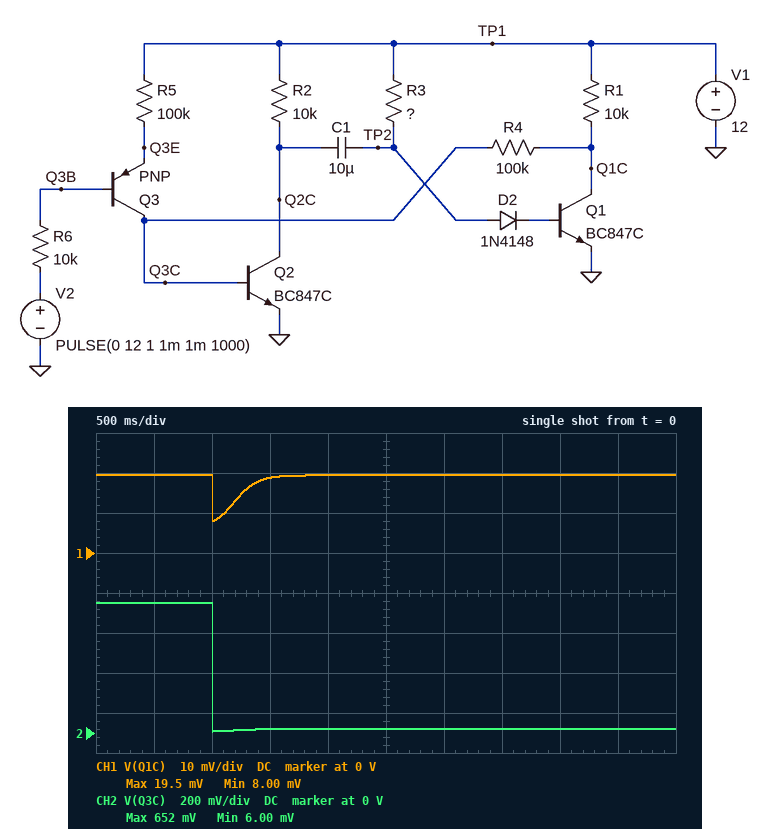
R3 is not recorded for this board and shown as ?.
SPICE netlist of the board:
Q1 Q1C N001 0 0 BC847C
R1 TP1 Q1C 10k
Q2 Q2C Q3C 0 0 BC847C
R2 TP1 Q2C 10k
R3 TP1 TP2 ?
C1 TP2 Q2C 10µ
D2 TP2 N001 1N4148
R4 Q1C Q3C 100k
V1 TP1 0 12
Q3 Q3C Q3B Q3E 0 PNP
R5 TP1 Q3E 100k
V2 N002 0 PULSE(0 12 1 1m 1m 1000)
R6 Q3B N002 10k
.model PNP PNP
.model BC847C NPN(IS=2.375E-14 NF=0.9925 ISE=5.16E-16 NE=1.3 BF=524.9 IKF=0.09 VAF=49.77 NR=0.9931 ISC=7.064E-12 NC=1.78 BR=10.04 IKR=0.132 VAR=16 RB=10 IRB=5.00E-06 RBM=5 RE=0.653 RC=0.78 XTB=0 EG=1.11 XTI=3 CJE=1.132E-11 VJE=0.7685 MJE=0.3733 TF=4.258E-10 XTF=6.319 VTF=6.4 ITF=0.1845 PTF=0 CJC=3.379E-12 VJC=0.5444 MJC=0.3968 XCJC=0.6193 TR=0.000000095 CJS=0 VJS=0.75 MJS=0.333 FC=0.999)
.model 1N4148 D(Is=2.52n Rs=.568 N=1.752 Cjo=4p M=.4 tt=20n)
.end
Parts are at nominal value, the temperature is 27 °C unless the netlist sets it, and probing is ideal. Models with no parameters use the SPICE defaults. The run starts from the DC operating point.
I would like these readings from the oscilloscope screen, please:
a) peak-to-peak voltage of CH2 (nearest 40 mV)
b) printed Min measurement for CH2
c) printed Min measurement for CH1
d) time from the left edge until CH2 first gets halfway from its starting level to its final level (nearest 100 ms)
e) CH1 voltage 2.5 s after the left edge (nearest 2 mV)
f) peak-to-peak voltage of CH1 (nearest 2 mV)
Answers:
640 mV
6.00 mV
8.00 mV
1.0 s
20 mV
12 mV
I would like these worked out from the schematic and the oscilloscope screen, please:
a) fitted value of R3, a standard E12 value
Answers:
68 kΩ
